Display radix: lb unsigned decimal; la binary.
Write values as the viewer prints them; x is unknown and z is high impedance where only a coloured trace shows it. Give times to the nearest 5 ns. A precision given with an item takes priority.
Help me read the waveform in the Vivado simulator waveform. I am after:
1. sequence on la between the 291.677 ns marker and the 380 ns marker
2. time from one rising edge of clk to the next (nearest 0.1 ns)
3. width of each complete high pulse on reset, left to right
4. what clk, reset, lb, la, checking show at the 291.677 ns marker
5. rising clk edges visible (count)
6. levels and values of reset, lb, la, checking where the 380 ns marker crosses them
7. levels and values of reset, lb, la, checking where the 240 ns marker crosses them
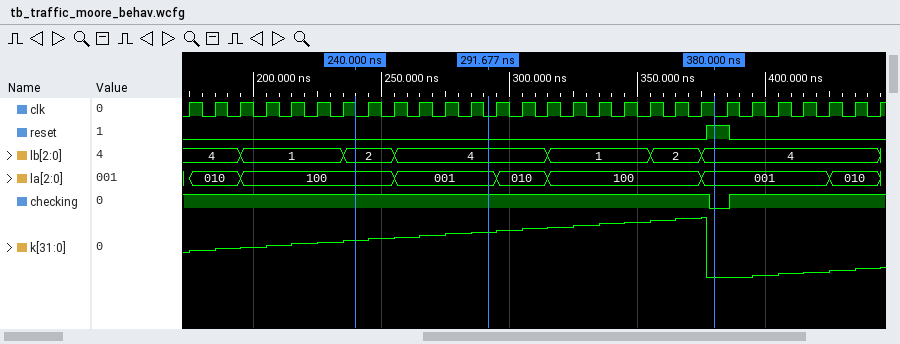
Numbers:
001, 010, 100, 001
10 ns
10 ns
clk=0, reset=0, lb=4, la=001, checking=1
28
reset=1, lb=4, la=001, checking=0
reset=0, lb=2, la=100, checking=1
